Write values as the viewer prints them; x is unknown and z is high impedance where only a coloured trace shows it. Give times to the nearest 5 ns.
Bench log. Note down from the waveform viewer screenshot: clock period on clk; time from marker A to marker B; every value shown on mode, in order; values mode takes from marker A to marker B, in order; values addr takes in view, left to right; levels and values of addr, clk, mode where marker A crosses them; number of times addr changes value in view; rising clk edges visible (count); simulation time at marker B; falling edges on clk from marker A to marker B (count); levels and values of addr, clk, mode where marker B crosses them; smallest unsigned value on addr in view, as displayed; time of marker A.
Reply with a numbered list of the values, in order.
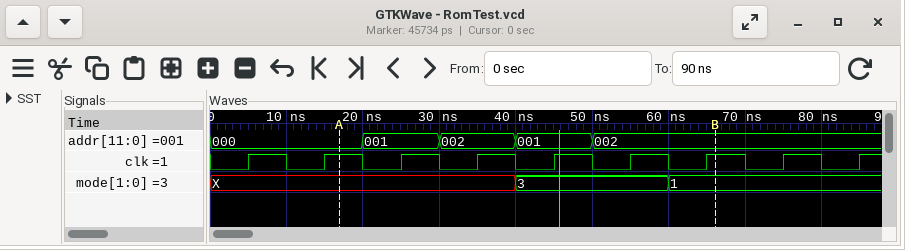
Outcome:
1. 10 ns
2. 50 ns
3. X, 3, 1
4. X, 3, 1
5. 000, 001, 002, 001, 002
6. addr=000, clk=1, mode=X
7. 4
8. 9
9. 65 ns
10. 5
11. addr=002, clk=1, mode=1
12. 000
13. 15 ns
